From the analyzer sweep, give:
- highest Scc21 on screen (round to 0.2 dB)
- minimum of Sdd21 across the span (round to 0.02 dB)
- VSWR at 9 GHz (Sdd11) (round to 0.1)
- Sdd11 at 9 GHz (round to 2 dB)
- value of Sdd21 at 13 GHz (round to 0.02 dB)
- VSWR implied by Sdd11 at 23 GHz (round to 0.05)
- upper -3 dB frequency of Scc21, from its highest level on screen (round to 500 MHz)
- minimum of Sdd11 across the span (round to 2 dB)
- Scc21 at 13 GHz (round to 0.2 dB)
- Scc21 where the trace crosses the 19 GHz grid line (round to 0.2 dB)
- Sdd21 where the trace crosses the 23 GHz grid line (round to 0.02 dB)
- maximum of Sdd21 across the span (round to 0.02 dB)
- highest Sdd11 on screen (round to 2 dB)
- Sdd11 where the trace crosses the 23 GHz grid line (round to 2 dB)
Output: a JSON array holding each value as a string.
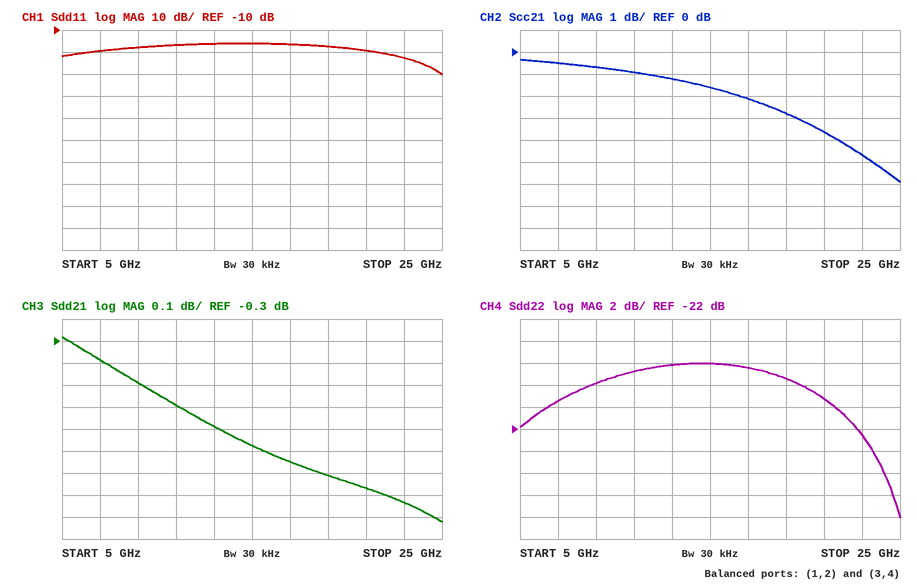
["-0.4 dB", "-1.12 dB", "1.3", "-18 dB", "-0.68 dB", "1.15", "20.5 GHz", "-30 dB", "-1.2 dB", "-2.8 dB", "-1.04 dB", "-0.28 dB", "-16 dB", "-22 dB"]
